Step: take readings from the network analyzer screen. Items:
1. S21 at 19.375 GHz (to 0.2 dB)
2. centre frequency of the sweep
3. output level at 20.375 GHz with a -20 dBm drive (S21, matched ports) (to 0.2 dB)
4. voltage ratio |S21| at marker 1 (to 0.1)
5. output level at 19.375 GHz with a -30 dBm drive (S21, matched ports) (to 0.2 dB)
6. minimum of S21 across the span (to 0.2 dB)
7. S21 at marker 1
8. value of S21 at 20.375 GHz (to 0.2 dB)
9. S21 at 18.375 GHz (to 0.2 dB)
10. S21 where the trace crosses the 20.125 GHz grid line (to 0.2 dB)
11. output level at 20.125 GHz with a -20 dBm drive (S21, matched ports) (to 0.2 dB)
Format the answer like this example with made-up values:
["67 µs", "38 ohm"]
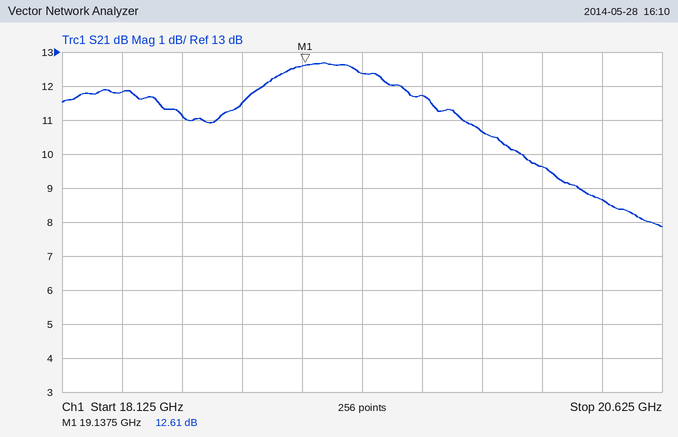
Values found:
["12.4 dB", "19.375 GHz", "-11.4 dBm", "4.3", "-17.6 dBm", "7.8 dB", "12.61 dB", "8.6 dB", "11.8 dB", "9.6 dB", "-10.4 dBm"]
